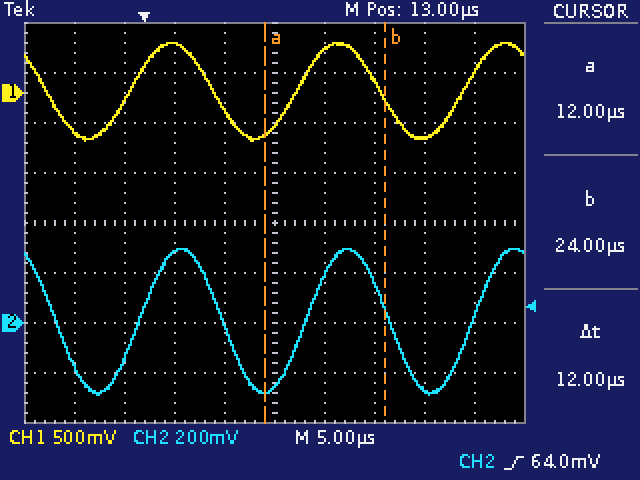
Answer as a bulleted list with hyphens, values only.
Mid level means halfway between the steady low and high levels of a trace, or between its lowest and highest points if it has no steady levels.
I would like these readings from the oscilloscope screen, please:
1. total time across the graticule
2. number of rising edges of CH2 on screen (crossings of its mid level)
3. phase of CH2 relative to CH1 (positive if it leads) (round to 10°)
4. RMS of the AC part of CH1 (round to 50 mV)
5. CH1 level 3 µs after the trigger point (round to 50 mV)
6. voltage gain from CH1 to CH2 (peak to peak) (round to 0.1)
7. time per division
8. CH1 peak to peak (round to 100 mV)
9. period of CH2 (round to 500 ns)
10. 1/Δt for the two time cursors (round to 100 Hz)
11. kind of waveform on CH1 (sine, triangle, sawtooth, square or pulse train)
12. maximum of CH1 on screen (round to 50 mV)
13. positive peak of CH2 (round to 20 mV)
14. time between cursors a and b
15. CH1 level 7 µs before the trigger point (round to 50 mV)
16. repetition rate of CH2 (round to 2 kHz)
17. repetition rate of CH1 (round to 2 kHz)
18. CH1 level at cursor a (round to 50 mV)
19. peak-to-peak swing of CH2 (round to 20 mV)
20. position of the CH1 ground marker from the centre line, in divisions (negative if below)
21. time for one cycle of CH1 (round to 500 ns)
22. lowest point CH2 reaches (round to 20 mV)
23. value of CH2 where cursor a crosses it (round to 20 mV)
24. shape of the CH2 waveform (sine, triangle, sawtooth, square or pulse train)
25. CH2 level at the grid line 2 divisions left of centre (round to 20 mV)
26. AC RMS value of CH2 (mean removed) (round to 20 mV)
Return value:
- 50 µs
- 3
- -20°
- 350 mV
- 500 mV
- 0.6
- 5 µs
- 1.00 V
- 16.5 µs
- 83.3 kHz
- sine
- 500 mV
- 300 mV
- 12 µs
- -400 mV
- 60 kHz
- 60 kHz
- -400 mV
- 580 mV
- +2.6 div
- 16.5 µs
- -280 mV
- -280 mV
- sine
- 280 mV
- 200 mV
